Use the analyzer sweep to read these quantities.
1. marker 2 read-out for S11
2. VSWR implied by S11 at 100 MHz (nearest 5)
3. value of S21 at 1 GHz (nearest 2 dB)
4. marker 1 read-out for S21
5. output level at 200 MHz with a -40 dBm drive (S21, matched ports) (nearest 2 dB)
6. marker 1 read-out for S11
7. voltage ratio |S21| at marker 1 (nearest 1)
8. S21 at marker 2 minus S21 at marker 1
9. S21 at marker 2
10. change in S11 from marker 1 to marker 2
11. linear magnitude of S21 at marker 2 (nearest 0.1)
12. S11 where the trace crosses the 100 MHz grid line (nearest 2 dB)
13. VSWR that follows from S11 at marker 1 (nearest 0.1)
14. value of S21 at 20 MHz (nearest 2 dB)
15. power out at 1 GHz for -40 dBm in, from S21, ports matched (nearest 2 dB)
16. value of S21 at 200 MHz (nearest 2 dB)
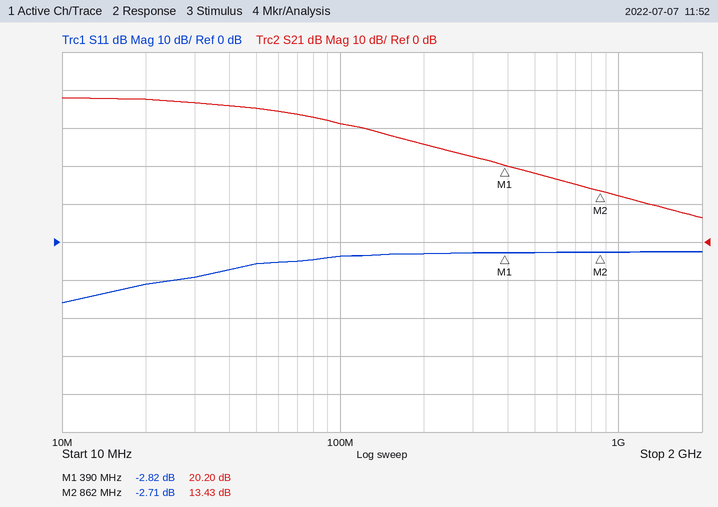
-2.71 dB
5
12 dB
20.20 dB
-14 dBm
-2.82 dB
10
-6.77 dB
13.43 dB
0.11 dB
4.7
-4 dB
6.2
38 dB
-28 dBm
26 dB
